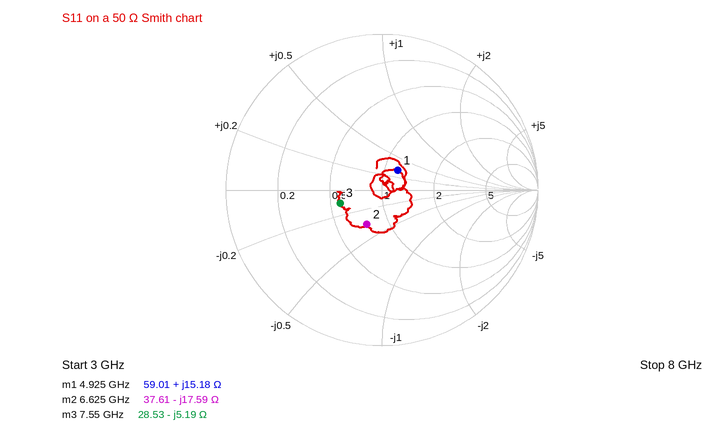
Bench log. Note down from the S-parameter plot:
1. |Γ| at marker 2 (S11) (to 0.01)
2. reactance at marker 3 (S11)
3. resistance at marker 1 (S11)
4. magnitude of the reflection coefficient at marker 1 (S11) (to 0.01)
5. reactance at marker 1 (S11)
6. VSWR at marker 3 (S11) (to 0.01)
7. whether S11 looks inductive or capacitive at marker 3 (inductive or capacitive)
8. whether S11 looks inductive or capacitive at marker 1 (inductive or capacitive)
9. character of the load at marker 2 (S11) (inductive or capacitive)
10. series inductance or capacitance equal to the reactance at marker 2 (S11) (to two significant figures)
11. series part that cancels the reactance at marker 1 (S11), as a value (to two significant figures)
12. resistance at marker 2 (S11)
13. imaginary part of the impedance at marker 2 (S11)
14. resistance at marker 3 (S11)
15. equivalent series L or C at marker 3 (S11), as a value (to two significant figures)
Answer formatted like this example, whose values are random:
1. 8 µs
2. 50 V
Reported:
1. 0.24
2. -5.19 Ω
3. 59.01 Ω
4. 0.16
5. +15.18 Ω
6. 1.78
7. capacitive
8. inductive
9. capacitive
10. 1.4 pF
11. 2.1 pF
12. 37.61 Ω
13. -17.59 Ω
14. 28.53 Ω
15. 4.1 pF
